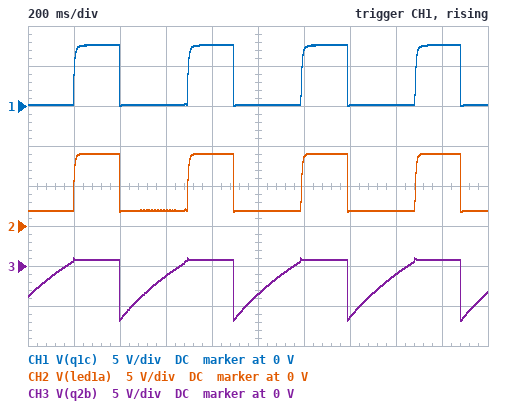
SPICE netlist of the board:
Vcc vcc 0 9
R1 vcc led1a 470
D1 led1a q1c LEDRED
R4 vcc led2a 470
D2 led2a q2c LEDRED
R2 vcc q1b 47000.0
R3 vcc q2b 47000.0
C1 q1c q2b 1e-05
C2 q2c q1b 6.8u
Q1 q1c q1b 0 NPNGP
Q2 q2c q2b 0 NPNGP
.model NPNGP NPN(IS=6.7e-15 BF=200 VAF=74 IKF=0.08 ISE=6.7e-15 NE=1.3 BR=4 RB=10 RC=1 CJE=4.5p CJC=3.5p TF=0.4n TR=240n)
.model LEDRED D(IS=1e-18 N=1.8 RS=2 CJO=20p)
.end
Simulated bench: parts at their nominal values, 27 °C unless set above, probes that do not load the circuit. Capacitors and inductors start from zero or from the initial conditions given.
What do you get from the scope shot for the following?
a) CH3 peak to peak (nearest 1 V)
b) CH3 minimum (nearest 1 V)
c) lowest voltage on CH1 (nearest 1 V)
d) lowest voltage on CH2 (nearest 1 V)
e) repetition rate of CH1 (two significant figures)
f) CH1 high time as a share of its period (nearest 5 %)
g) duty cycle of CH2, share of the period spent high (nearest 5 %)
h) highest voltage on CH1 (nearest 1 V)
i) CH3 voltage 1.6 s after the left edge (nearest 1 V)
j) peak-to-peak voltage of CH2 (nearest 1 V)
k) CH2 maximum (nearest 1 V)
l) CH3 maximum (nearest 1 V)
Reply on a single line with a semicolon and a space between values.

8 V; -7 V; 0 V; 2 V; 2.0 Hz; 40 %; 40 %; 8 V; -1 V; 7 V; 9 V; 1 V
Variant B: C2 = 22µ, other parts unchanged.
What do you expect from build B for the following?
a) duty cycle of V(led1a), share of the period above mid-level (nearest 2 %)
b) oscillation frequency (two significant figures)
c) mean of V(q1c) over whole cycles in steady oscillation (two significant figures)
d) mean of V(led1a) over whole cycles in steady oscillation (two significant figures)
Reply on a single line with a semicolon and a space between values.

68 %; 1.1 Hz; 5.3 V; 6.7 V
